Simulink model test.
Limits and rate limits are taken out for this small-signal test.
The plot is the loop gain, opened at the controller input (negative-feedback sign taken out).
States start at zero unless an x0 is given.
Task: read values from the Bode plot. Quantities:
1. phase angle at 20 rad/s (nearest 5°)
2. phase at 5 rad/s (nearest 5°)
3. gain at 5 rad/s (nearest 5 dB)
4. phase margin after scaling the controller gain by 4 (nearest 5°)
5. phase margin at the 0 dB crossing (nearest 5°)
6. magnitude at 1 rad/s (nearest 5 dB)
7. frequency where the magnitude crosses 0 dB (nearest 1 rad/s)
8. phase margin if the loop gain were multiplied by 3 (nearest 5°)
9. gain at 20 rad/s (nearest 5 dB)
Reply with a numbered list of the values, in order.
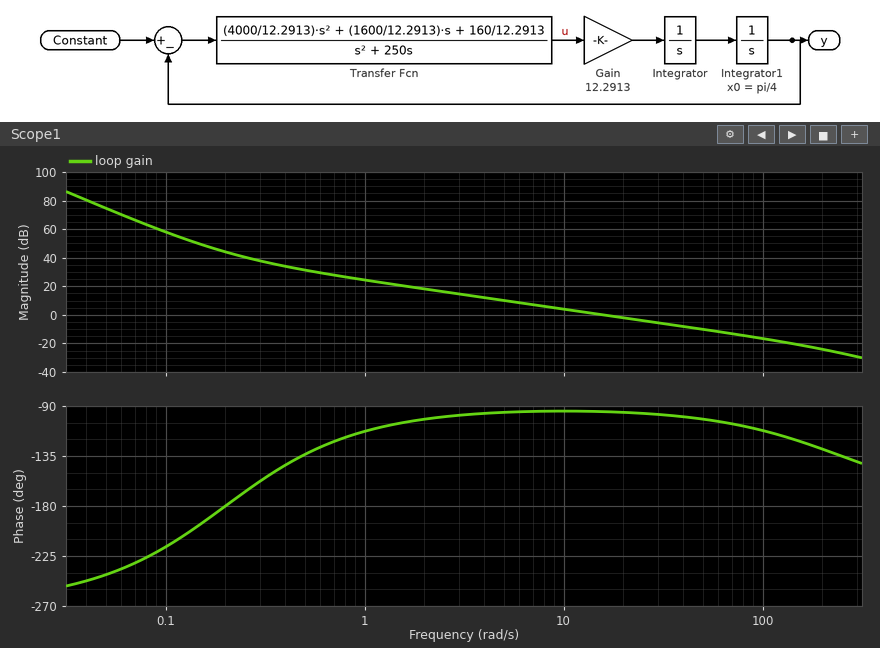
1. -95°
2. -95°
3. 10 dB
4. 75°
5. 85°
6. 25 dB
7. 16 rad/s
8. 80°
9. 0 dB
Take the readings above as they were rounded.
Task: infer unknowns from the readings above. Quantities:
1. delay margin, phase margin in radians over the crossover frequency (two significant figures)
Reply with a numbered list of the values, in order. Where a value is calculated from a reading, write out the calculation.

1. 85 × π / 180 / 16 = 0.093 s
